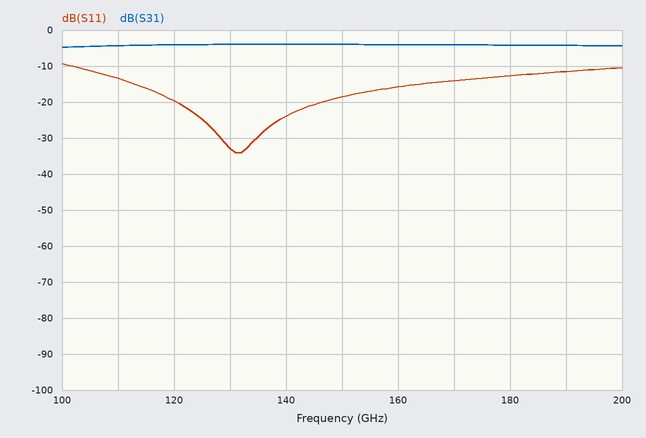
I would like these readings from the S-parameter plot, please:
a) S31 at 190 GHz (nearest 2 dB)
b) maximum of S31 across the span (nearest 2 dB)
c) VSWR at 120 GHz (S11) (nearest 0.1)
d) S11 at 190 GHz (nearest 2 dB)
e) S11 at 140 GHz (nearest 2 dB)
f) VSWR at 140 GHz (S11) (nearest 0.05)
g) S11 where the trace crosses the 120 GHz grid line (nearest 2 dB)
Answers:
-4 dB
-4 dB
1.2
-12 dB
-24 dB
1.15
-20 dB
